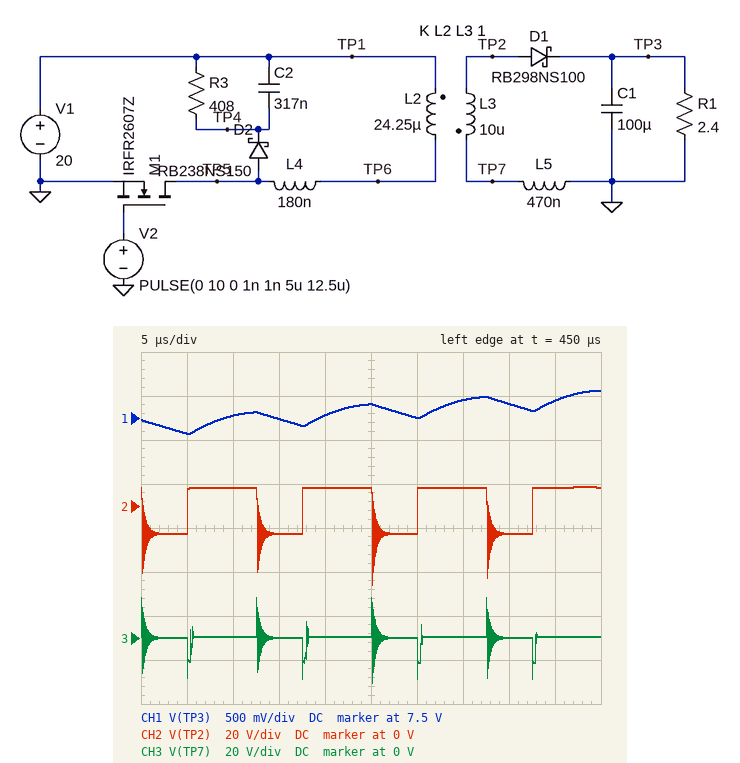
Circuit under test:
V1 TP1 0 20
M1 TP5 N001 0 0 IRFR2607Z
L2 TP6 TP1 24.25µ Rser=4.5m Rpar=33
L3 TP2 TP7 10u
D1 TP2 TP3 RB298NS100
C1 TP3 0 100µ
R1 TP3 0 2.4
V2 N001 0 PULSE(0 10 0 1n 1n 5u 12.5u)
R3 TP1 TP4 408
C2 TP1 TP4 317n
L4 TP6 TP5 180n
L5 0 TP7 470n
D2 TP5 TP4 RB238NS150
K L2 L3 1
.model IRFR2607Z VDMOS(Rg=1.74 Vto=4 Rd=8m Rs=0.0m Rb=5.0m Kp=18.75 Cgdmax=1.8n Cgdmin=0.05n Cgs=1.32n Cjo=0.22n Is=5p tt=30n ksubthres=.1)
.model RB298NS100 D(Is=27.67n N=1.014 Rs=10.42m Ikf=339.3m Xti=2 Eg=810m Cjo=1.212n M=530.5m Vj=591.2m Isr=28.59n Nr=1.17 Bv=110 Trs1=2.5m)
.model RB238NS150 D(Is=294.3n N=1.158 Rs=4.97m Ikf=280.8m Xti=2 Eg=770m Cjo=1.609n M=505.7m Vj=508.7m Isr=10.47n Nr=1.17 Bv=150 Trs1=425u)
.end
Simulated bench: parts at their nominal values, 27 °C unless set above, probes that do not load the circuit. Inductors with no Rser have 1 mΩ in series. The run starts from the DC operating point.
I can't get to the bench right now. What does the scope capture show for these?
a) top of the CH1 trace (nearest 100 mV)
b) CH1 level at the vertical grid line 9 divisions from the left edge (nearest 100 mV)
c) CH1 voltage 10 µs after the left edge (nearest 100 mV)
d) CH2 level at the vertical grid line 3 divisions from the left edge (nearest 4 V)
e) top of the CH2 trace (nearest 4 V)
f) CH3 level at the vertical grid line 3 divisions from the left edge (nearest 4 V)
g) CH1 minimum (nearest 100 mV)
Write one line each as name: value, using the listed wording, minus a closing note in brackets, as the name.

top of the CH1 trace: 7.8 V
CH1 level at the vertical grid line 9 divisions from the left edge: 7.7 V
CH1 voltage 10 µs after the left edge: 7.5 V
CH2 level at the vertical grid line 3 divisions from the left edge: -12 V
top of the CH2 trace: 8 V
CH3 level at the vertical grid line 3 divisions from the left edge: 0 V
CH1 minimum: 7.3 V
